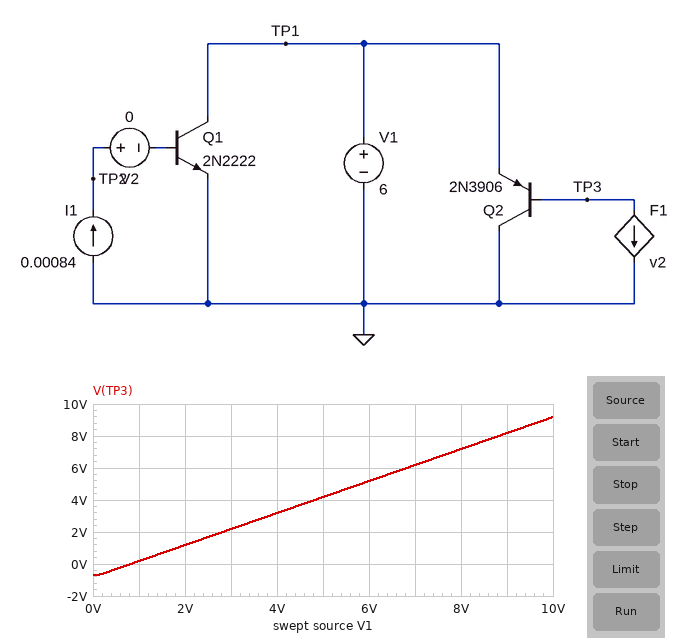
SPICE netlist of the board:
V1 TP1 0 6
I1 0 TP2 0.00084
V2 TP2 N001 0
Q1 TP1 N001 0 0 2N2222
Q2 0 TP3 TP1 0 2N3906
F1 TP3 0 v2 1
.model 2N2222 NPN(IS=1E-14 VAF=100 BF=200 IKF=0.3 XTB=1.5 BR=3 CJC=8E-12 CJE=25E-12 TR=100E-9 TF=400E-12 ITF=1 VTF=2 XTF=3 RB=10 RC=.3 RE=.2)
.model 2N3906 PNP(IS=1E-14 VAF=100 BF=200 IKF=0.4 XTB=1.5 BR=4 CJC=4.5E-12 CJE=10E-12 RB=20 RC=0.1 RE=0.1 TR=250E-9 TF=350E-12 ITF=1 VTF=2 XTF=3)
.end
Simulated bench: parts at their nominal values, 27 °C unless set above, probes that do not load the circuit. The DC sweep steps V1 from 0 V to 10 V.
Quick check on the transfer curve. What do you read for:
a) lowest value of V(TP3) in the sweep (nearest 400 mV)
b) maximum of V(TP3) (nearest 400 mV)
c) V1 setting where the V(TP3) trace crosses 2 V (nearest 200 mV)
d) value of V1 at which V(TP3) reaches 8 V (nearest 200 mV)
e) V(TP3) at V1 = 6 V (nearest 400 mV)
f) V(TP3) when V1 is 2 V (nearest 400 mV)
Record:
-800 mV
9.2 V
2.8 V
8.8 V
5.2 V
1.2 V
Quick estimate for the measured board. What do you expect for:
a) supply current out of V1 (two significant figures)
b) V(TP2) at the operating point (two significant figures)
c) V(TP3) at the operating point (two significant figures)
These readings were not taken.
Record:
260 mA
820 mV
5.2 V
